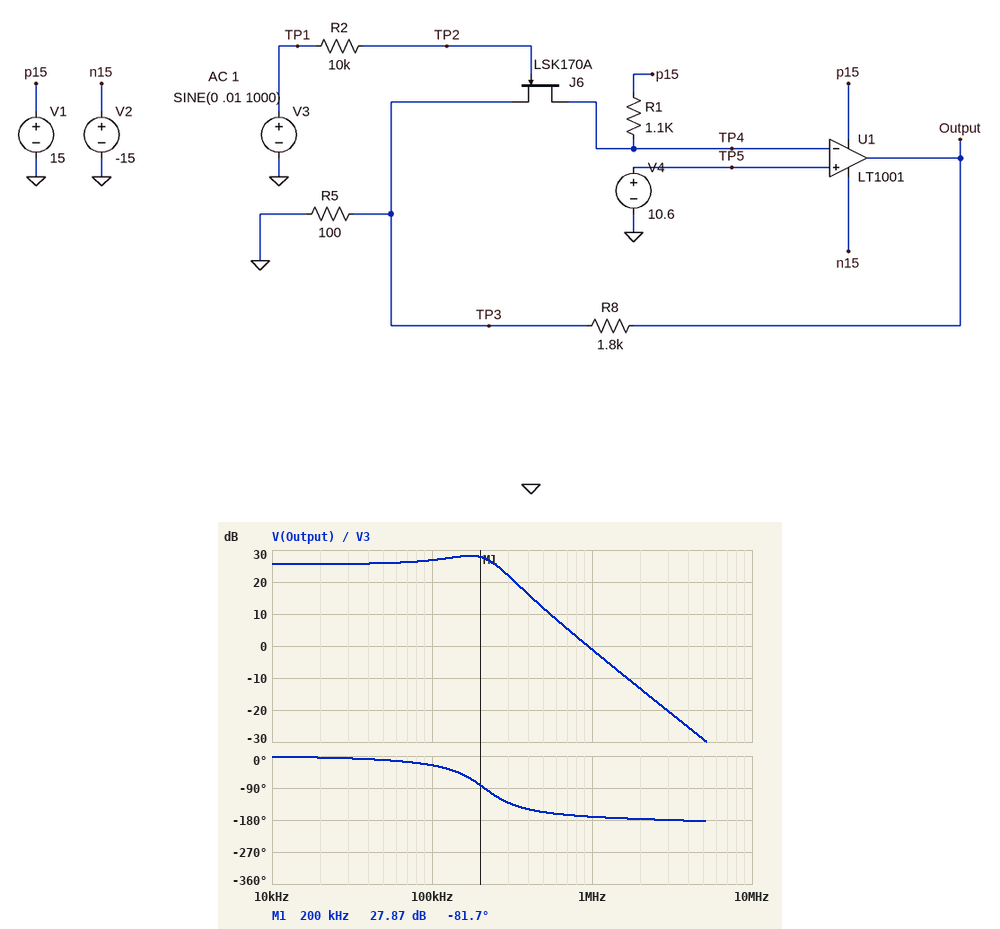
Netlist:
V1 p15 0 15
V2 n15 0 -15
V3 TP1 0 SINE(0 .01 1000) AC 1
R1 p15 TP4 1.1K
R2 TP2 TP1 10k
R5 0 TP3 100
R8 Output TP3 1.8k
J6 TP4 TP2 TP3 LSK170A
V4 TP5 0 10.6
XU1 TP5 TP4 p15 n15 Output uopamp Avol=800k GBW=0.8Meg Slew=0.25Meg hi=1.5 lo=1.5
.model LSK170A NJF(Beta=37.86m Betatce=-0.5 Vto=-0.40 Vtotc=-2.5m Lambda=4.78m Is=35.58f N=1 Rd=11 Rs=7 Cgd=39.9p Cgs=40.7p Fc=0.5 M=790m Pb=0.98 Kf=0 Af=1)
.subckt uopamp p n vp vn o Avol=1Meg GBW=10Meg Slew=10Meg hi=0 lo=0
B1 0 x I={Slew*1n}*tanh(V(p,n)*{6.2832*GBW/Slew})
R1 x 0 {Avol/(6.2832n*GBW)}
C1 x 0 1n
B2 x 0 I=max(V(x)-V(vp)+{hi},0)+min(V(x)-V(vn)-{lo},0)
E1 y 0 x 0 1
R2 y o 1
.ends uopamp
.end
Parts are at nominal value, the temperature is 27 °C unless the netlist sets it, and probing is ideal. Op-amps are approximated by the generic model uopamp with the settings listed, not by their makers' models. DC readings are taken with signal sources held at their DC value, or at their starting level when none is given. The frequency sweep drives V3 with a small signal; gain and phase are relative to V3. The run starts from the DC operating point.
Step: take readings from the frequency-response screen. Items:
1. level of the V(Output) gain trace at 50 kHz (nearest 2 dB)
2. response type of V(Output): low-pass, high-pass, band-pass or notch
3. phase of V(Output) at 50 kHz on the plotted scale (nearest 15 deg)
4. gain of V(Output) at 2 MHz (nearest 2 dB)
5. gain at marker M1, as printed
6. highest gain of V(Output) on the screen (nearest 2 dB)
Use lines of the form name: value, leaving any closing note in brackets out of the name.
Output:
level of the V(Output) gain trace at 50 kHz: 26 dB
response type of V(Output): low-pass, high-pass, band-pass or notch: low-pass
phase of V(Output) at 50 kHz on the plotted scale: -15 deg
gain of V(Output) at 2 MHz: -14 dB
gain at marker M1, as printed: 27.87 dB
highest gain of V(Output) on the screen: 28 dB
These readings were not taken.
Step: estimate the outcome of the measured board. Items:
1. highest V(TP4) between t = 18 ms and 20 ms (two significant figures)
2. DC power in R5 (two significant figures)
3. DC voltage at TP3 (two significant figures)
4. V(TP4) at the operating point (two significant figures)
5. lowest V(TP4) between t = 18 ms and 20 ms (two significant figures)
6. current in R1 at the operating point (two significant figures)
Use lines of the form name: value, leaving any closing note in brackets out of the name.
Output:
highest V(TP4) between t = 18 ms and 20 ms: 11 V
DC power in R5: 30 µW
DC voltage at TP3: 55 mV
V(TP4) at the operating point: 11 V
lowest V(TP4) between t = 18 ms and 20 ms: 11 V
current in R1 at the operating point: 4.0 mA
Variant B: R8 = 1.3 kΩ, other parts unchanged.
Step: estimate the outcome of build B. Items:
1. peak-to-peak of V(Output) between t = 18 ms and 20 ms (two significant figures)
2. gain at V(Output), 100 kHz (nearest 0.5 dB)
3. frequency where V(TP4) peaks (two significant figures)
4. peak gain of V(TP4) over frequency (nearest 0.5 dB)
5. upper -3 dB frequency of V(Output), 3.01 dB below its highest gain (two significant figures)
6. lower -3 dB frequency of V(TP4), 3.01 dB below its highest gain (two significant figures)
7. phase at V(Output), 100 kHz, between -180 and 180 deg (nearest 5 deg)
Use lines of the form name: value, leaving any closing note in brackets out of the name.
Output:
peak-to-peak of V(Output) between t = 18 ms and 20 ms: 280 mV
gain at V(Output), 100 kHz: 24.0 dB
frequency where V(TP4) peaks: 250 kHz
peak gain of V(TP4) over frequency: 15.5 dB
upper -3 dB frequency of V(Output), 3.01 dB below its highest gain: 290 kHz
lower -3 dB frequency of V(TP4), 3.01 dB below its highest gain: 170 kHz
phase at V(Output), 100 kHz, between -180 and 180 deg: -20 deg
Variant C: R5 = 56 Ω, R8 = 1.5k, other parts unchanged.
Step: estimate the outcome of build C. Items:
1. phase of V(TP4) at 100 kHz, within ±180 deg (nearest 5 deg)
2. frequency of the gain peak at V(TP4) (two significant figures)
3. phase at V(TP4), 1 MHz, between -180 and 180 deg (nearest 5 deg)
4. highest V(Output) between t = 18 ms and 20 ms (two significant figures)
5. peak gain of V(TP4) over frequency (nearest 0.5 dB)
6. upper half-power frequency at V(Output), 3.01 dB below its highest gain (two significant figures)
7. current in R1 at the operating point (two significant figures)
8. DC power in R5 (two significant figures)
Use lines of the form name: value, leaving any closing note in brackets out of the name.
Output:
phase of V(TP4) at 100 kHz, within ±180 deg: -120 deg
frequency of the gain peak at V(TP4): 180 kHz
phase at V(TP4), 1 MHz, between -180 and 180 deg: 95 deg
highest V(Output) between t = 18 ms and 20 ms: -4.2 V
peak gain of V(TP4) over frequency: 19.0 dB
upper half-power frequency at V(Output), 3.01 dB below its highest gain: 210 kHz
current in R1 at the operating point: 4.0 mA
DC power in R5: 54 µW
